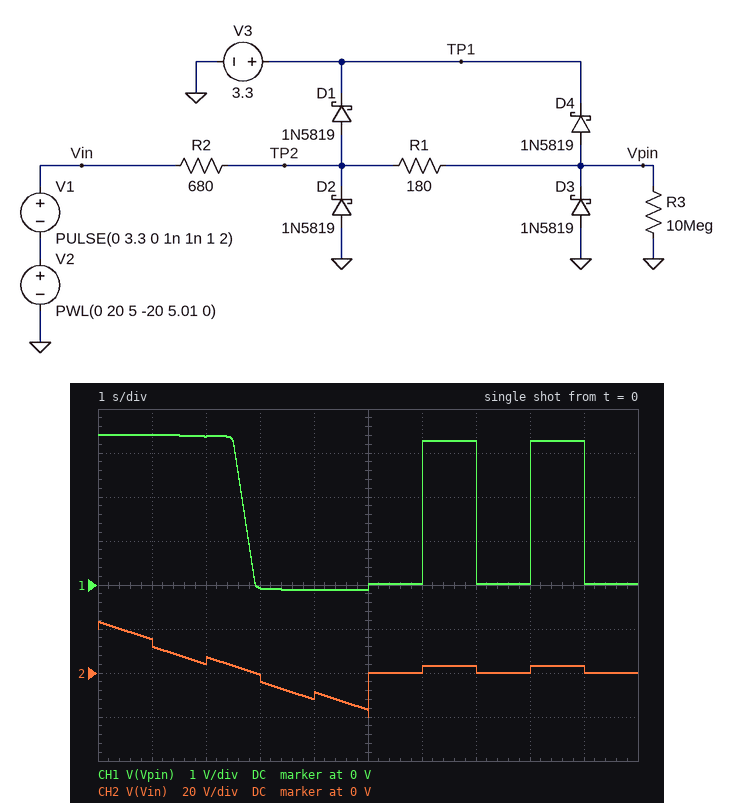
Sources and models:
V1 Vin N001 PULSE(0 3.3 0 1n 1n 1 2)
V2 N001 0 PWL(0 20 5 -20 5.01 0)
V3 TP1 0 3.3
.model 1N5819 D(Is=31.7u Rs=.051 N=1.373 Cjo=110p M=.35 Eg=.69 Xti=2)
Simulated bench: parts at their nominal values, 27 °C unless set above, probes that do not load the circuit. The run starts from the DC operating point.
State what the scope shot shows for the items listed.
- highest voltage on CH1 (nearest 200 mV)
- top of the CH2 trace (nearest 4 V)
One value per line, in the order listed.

3.4 V
24 V
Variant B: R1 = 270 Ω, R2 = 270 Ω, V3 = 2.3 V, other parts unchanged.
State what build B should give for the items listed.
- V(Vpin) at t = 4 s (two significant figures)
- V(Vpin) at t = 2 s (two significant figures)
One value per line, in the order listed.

-100 mV
2.4 V
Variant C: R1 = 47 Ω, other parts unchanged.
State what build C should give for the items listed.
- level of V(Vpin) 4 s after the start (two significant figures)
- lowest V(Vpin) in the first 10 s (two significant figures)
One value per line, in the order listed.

-140 mV
-150 mV
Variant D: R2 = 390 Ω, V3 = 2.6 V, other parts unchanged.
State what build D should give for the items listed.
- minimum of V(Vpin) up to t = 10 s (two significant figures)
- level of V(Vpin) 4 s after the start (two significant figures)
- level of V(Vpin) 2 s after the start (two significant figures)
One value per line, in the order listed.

-120 mV
-110 mV
2.7 V
